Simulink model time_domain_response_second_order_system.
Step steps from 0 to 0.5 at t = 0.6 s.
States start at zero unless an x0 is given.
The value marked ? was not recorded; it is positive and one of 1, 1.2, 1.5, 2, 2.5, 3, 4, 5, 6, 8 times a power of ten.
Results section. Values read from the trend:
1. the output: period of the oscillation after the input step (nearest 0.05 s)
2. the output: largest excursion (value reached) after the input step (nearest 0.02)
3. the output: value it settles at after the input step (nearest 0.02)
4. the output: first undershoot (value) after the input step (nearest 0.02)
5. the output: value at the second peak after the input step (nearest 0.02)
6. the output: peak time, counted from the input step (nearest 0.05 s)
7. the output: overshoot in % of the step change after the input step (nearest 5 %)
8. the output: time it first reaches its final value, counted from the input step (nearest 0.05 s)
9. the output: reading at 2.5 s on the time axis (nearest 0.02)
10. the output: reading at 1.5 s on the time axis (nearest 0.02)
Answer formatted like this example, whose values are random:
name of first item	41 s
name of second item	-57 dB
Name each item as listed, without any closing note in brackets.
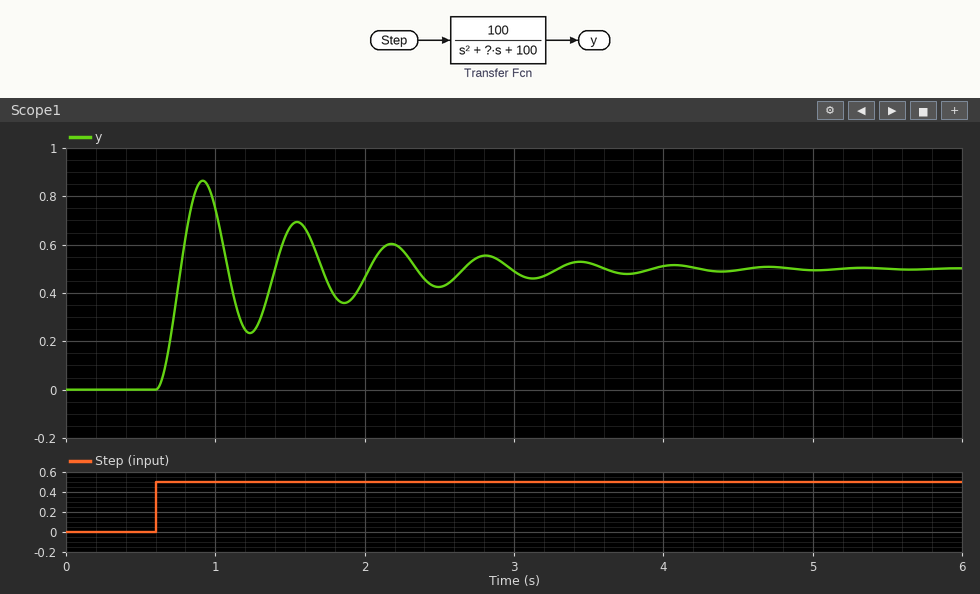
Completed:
the output: period of the oscillation after the input step	0.65 s
the output: largest excursion (value reached) after the input step	0.86
the output: value it settles at after the input step	0.50
the output: first undershoot (value) after the input step	0.24
the output: value at the second peak after the input step	0.70
the output: peak time, counted from the input step	0.30 s
the output: overshoot in % of the step change after the input step	75 %
the output: time it first reaches its final value, counted from the input step	0.15 s
the output: reading at 2.5 s on the time axis	0.42
the output: reading at 1.5 s on the time axis	0.68
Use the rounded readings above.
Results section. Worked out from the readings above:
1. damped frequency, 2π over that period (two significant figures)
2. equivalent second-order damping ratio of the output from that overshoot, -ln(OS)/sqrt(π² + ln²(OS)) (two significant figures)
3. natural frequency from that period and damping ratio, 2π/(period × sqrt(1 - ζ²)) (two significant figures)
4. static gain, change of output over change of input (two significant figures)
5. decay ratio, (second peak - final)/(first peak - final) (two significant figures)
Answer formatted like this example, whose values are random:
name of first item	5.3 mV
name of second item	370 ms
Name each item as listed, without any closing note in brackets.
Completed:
damped frequency, 2π over that period	9.7 rad/s
equivalent second-order damping ratio of the output from that overshoot, -ln(OS)/sqrt(π² + ln²(OS))	0.091
natural frequency from that period and damping ratio, 2π/(period × sqrt(1 - ζ²))	9.7 rad/s
static gain, change of output over change of input	1.0
decay ratio, (second peak - final)/(first peak - final)	0.56
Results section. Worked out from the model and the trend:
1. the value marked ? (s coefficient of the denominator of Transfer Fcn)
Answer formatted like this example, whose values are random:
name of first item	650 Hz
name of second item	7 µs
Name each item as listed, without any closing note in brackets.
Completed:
the value marked ?	2
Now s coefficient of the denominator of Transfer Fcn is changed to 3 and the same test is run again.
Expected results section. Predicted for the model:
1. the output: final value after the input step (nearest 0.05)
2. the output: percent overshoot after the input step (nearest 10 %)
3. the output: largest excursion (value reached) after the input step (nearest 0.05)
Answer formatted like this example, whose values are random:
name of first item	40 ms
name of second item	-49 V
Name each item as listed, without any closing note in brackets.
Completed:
the output: final value after the input step	0.50
the output: percent overshoot after the input step	60 %
the output: largest excursion (value reached) after the input step	0.80
